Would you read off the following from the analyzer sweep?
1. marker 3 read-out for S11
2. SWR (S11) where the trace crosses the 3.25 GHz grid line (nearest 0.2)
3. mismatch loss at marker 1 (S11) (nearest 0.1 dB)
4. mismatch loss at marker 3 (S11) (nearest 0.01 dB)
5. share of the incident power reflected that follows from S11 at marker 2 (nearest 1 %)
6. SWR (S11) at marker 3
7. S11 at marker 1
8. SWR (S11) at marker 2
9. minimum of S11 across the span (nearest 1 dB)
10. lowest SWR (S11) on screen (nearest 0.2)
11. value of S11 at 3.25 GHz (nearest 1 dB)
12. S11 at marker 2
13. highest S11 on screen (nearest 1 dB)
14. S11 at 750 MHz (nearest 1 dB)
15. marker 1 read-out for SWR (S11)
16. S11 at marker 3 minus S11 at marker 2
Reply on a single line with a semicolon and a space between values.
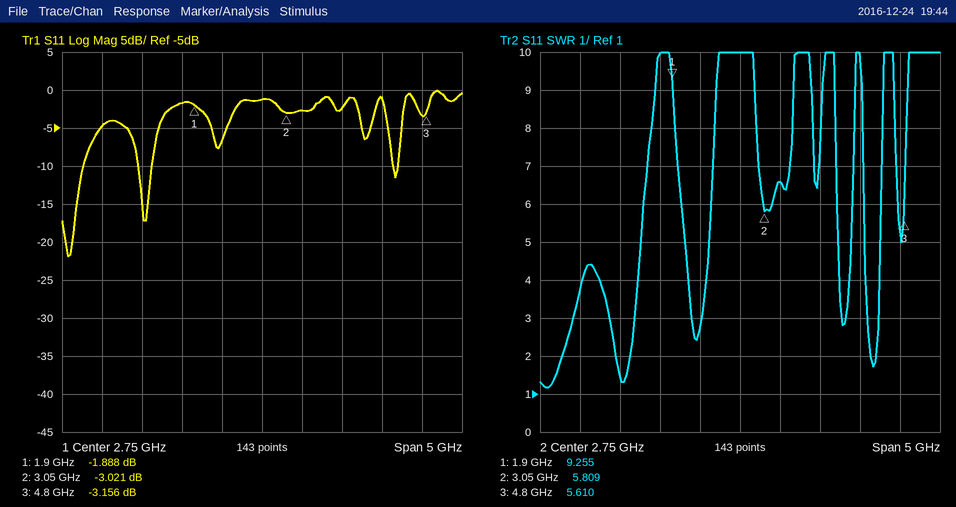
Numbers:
-3.156 dB; 6.6; 4.5 dB; 2.87 dB; 50 %; 5.610; -1.888 dB; 5.809; -22 dB; 1.2; -3 dB; -3.021 dB; 0 dB; -5 dB; 9.255; -0.135 dB
